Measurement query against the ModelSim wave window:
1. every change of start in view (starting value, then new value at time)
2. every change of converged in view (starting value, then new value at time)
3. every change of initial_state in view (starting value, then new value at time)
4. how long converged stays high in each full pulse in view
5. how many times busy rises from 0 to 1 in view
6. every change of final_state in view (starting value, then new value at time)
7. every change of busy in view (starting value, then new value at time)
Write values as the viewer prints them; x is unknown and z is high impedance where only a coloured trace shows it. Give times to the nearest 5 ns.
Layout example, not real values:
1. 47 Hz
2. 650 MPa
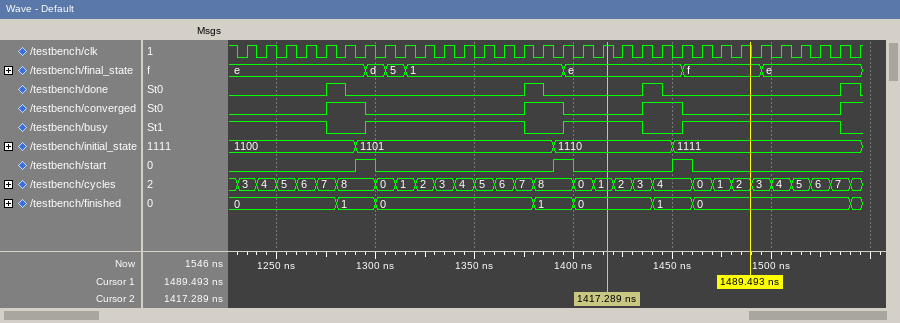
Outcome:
1. 0, 1 at 1290 ns, 0 at 1300 ns, 1 at 1390 ns, 0 at 1400 ns, 1 at 1450 ns, 0 at 1460 ns
2. 0, 1 at 1275 ns, 0 at 1295 ns, 1 at 1375 ns, 0 at 1395 ns, 1 at 1435 ns, 0 at 1455 ns, 1 at 1535 ns
3. 1100, 1101 at 1290 ns, 1110 at 1390 ns, 1111 at 1450 ns
4. 20 ns, 20 ns, 20 ns
5. 3
6. e, d at 1295 ns, 5 at 1305 ns, 1 at 1315 ns, e at 1395 ns, f at 1455 ns, e at 1495 ns
7. 1, 0 at 1275 ns, 1 at 1295 ns, 0 at 1375 ns, 1 at 1395 ns, 0 at 1435 ns, 1 at 1455 ns, 0 at 1535 ns
